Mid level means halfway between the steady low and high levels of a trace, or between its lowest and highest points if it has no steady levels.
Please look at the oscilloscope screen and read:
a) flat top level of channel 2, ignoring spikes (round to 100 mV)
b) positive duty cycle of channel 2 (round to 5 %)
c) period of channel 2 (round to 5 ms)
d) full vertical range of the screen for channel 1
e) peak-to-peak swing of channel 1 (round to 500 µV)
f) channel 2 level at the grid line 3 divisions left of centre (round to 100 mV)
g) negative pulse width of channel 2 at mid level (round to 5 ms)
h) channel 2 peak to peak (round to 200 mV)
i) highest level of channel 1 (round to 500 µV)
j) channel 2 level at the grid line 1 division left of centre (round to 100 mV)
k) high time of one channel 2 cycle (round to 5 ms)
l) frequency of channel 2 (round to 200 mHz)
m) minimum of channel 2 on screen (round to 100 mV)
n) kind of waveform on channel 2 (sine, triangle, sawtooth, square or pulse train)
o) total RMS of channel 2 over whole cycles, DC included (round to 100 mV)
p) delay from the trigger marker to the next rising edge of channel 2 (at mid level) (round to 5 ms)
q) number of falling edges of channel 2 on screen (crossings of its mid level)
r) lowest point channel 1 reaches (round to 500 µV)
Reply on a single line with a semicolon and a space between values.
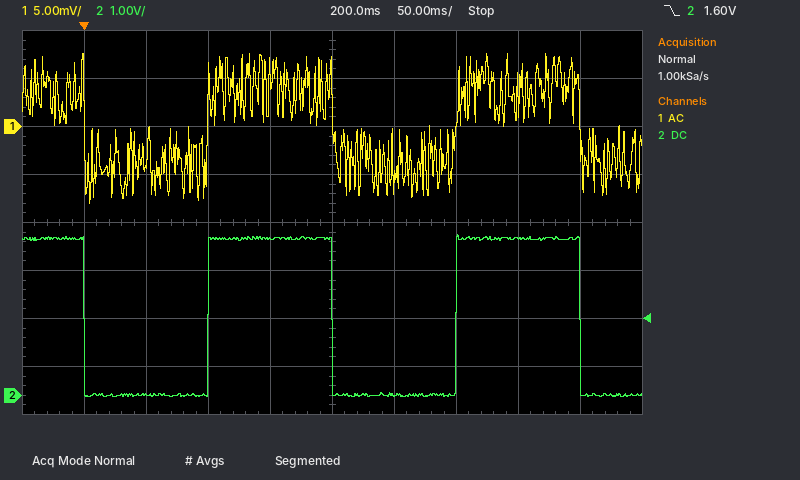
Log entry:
3.3 V; 50 %; 200 ms; 40 mV; 15.5 mV; 0.0 V; 100 ms; 3.4 V; 7.5 mV; 3.3 V; 100 ms; 5.0 Hz; 0.0 V; square; 2.3 V; 100 ms; 3; -8.0 mV
